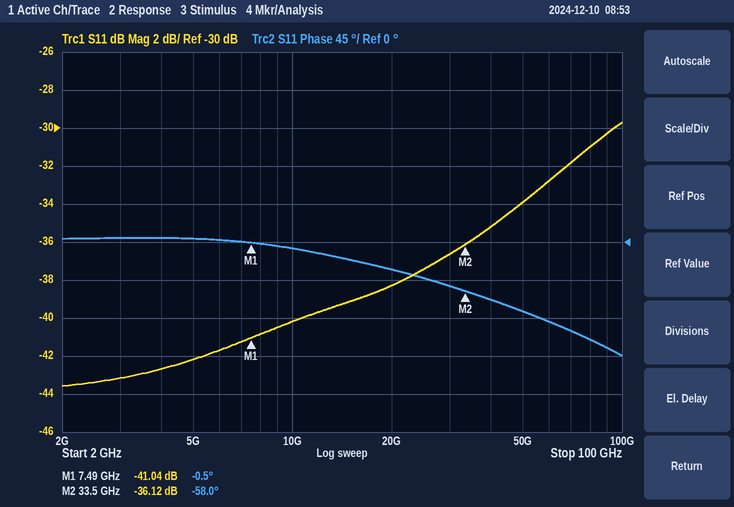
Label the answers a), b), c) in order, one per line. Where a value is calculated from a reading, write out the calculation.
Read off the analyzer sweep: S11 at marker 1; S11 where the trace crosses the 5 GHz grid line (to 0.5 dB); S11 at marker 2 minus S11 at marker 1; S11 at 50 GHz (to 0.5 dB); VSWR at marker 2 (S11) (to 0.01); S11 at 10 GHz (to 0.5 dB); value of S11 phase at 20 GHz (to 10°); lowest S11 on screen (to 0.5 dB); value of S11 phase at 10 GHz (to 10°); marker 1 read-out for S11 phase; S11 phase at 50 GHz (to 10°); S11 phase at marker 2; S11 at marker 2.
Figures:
a) -41.04 dB
b) -42.0 dB
c) -36.12 − (-41.04) = 4.92 dB
d) -34.0 dB
e) (1 + 0.0156)/(1 − 0.0156) ≈ 1.03
f) -40.0 dB
g) -30°
h) -43.5 dB
i) -10°
j) -0.5°
k) -80°
l) -58.0°
m) -36.12 dB
